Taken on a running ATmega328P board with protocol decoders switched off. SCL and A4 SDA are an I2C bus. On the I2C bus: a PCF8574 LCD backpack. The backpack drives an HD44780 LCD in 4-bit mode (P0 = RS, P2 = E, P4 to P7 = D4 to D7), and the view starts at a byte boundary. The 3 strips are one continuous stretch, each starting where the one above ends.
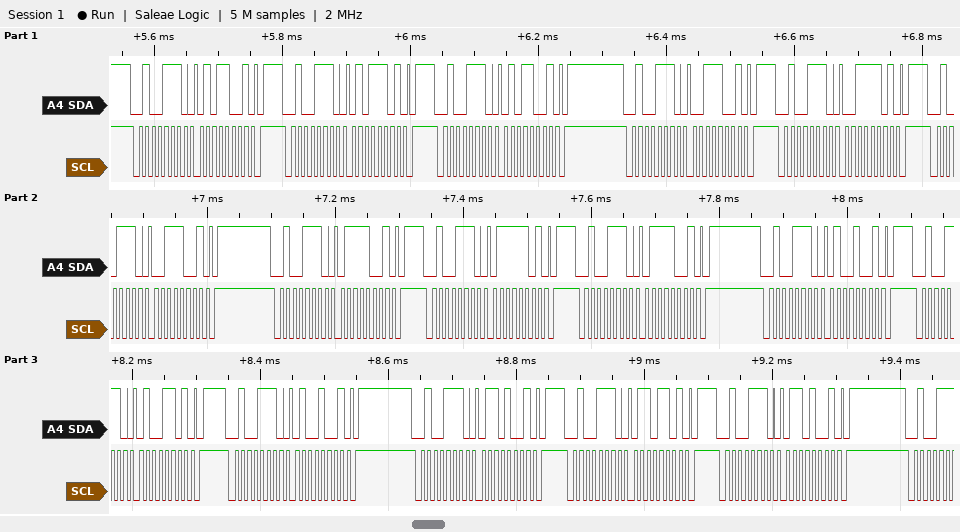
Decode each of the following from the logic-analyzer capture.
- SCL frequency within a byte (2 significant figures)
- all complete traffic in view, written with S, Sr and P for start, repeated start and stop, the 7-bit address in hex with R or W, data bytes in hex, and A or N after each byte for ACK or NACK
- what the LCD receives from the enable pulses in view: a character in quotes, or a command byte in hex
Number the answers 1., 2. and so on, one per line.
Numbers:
1. 100 kHz
2. S 27W A 59 A P S 27W A 5D A P S 27W A 59 A P S 27W A 39 A P S 27W A 3D A P S 27W A 39 A P S 27W A 79 A P S 27W A 7D A P S 27W A 79 A P S 27W A 49 A P S 27W A 4D A P S 27W A 49 A P S 27W A 69 A P S 27W A 6D A P S 27W A 69 A P
3. 'S' 't'
